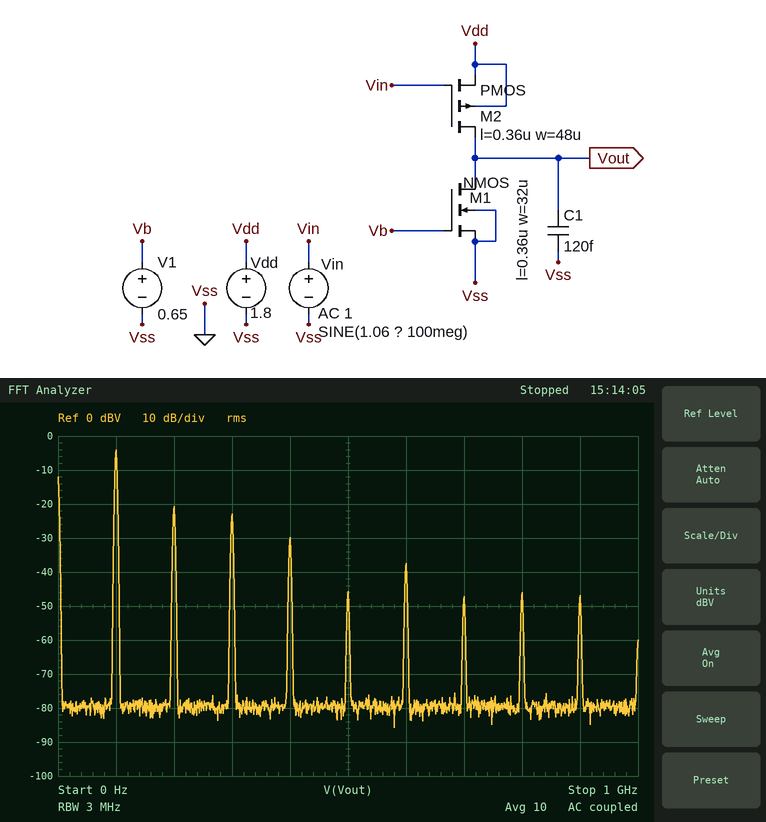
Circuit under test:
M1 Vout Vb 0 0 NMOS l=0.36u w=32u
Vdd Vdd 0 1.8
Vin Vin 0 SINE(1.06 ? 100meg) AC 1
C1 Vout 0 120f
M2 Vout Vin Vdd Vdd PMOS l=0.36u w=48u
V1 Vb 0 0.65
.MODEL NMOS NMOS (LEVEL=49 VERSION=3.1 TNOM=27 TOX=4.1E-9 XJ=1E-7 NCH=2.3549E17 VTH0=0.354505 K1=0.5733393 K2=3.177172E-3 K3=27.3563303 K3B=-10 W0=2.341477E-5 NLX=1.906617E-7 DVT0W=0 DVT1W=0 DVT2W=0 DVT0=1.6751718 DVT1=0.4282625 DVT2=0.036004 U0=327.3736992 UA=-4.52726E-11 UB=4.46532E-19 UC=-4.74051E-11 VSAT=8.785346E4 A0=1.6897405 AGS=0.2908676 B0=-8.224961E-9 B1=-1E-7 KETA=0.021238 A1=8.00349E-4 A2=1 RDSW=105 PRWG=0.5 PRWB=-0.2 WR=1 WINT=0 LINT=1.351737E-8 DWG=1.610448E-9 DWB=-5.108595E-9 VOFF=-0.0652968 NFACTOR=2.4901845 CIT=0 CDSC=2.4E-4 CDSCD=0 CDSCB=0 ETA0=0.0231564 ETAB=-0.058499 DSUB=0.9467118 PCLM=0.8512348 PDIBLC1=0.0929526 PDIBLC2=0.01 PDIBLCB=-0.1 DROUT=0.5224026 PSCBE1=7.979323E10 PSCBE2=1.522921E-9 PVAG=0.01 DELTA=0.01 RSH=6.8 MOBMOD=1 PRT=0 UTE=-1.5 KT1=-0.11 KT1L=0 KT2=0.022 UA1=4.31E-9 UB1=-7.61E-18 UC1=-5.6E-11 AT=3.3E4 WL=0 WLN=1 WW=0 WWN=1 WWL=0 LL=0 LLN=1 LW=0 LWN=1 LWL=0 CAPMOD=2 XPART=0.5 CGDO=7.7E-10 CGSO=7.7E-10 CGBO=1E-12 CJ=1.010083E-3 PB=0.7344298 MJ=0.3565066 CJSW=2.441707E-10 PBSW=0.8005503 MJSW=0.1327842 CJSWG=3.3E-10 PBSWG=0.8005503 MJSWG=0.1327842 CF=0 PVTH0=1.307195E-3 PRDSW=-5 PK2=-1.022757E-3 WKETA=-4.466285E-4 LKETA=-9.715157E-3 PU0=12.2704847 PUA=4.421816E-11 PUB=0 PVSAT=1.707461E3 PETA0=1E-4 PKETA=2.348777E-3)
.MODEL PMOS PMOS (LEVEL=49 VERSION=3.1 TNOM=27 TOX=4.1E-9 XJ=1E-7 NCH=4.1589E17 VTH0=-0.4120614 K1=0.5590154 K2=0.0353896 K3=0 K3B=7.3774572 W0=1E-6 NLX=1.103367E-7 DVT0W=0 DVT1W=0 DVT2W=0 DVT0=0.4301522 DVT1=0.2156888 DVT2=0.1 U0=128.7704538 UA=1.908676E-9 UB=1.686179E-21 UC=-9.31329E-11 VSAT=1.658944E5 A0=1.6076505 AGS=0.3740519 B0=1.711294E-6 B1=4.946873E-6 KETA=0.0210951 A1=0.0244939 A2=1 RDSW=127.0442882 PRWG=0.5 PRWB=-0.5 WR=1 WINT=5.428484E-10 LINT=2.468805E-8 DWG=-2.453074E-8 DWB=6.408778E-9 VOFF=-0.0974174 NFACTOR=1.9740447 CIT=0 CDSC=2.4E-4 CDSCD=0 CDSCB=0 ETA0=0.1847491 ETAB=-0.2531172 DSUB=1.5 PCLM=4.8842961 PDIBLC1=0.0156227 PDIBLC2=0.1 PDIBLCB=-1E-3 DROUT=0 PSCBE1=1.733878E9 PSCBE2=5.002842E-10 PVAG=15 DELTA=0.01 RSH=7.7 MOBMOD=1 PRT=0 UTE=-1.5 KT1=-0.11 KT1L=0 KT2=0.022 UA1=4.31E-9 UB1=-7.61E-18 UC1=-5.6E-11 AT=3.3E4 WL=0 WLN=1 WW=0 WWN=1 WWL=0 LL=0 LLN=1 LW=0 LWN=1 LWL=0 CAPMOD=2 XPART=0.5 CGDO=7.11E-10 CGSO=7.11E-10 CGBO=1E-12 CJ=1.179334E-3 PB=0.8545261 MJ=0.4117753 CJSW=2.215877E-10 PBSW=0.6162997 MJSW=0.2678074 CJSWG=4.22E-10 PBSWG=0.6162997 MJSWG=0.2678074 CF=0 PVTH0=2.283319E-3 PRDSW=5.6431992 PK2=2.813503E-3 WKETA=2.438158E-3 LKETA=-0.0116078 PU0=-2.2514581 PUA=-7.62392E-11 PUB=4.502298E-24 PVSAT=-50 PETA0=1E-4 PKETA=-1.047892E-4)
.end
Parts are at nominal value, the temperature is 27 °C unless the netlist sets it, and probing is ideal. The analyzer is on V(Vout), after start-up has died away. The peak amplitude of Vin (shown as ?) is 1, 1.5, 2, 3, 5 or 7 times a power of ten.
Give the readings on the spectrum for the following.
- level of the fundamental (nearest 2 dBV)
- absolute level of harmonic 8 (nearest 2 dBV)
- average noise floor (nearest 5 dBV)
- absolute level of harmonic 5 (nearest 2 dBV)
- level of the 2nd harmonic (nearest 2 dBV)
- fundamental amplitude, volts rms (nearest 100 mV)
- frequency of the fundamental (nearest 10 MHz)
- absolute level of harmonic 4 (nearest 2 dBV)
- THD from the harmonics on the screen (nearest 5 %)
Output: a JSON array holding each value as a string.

["-4 dBV", "-46 dBV", "-80 dBV", "-46 dBV", "-20 dBV", "600 mV", "100 MHz", "-30 dBV", "20 %"]
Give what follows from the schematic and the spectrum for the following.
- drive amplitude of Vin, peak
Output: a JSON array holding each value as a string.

["100 mV"]
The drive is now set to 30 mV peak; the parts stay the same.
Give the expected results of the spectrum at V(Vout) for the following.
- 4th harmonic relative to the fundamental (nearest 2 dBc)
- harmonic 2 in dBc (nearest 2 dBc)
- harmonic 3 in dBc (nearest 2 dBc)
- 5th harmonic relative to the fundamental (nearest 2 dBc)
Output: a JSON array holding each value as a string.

["-36 dBc", "-20 dBc", "-28 dBc", "-44 dBc"]
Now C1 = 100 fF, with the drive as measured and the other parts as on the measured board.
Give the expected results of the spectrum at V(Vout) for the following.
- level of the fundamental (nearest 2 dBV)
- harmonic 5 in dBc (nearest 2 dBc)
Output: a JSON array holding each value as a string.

["-4 dBV", "-40 dBc"]
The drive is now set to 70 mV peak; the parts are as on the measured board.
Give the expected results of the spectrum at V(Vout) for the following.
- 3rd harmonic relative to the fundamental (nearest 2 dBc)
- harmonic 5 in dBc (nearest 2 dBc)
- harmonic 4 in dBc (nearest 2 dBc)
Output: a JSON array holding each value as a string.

["-24 dBc", "-38 dBc", "-30 dBc"]
